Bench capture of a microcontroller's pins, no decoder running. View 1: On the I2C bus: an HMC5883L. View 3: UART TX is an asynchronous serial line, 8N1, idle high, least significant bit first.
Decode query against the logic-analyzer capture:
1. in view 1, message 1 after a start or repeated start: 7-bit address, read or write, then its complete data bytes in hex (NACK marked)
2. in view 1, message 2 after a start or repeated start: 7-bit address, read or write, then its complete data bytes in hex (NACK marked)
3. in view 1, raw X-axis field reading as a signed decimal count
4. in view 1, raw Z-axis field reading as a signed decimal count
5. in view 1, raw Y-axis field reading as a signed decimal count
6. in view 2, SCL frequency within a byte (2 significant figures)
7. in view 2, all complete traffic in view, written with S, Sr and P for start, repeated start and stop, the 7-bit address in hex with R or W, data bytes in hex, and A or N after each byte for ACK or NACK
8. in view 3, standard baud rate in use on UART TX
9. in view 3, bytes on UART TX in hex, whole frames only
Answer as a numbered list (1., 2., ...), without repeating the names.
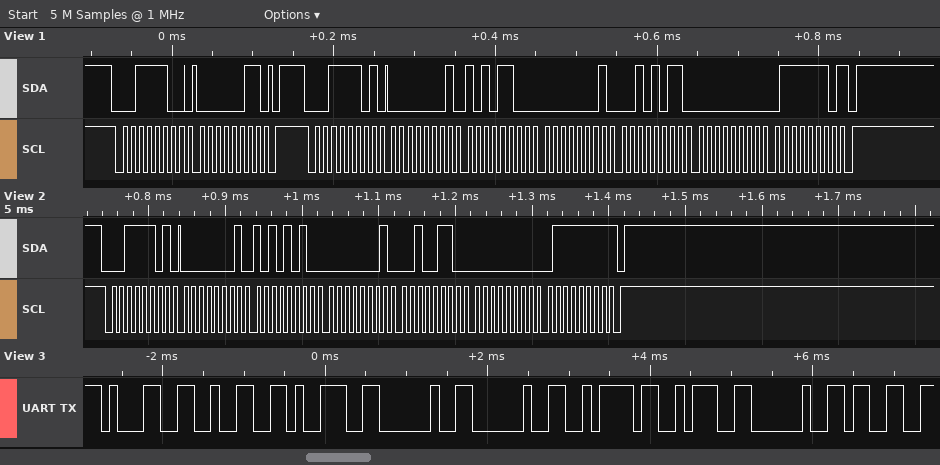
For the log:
1. 0x1E write: 03
2. 0x1E read: 01 AC 01 2B 00 7E NACK
3. 428
4. 299
5. 126
6. 100 kHz
7. S 1ER A 01 A AA A 01 A 26 A 00 A 7F N P
8. 9600 baud
9. 31 32 39 20 20 7A 3A 20 33
